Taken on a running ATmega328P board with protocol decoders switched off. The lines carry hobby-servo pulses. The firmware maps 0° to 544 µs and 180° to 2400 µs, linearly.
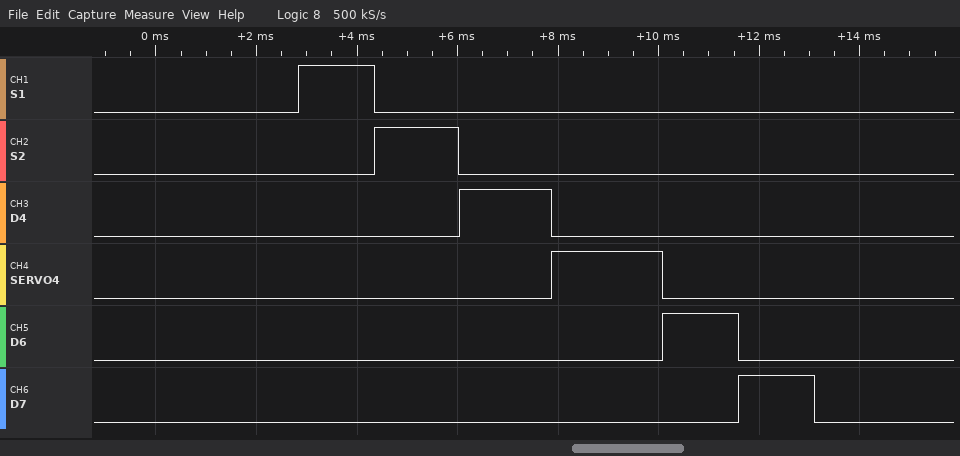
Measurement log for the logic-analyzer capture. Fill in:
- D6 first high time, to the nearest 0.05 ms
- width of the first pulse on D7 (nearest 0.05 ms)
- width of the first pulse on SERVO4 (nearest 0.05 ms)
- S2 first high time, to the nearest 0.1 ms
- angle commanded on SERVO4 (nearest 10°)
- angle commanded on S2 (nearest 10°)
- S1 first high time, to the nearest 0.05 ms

1.50 ms
1.50 ms
2.20 ms
1.7 ms
160°
110°
1.50 ms
